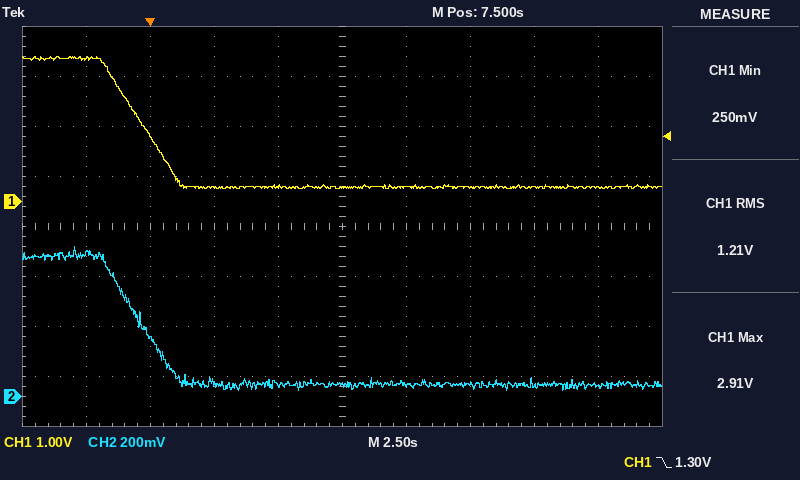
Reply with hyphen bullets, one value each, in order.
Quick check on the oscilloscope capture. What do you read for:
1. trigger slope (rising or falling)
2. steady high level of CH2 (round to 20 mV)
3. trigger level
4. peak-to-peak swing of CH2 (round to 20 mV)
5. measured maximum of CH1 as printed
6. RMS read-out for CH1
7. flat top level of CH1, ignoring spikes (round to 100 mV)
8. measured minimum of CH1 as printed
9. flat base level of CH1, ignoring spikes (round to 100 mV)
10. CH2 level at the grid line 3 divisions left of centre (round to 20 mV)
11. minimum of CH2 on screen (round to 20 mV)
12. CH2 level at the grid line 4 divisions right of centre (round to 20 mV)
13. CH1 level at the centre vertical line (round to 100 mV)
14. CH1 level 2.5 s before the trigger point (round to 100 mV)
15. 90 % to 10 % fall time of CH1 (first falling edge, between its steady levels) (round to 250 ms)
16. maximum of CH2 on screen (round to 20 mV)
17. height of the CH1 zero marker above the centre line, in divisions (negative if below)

- falling
- 560 mV
- 1.30 V
- 580 mV
- 2.91 V
- 1.21 V
- 2.9 V
- 250 mV
- 300 mV
- 240 mV
- 20 mV
- 40 mV
- 300 mV
- 2.9 V
- 2.50 s
- 600 mV
- +0.5 div
